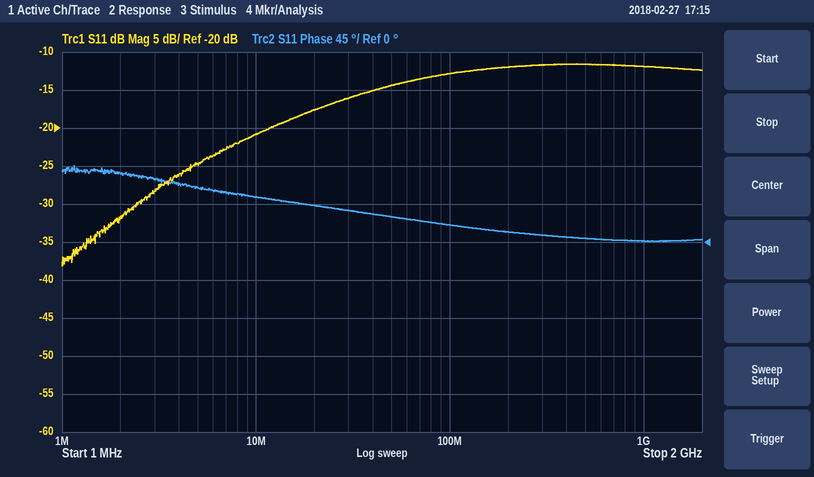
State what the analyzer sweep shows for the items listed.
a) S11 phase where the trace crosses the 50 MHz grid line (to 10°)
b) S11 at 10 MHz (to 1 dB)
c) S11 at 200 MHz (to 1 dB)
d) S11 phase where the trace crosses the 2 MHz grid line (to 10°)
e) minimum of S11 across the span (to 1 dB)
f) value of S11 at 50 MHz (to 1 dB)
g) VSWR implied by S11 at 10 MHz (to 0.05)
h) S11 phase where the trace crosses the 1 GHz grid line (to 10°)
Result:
30°
-21 dB
-12 dB
80°
-38 dB
-14 dB
1.20
0°
